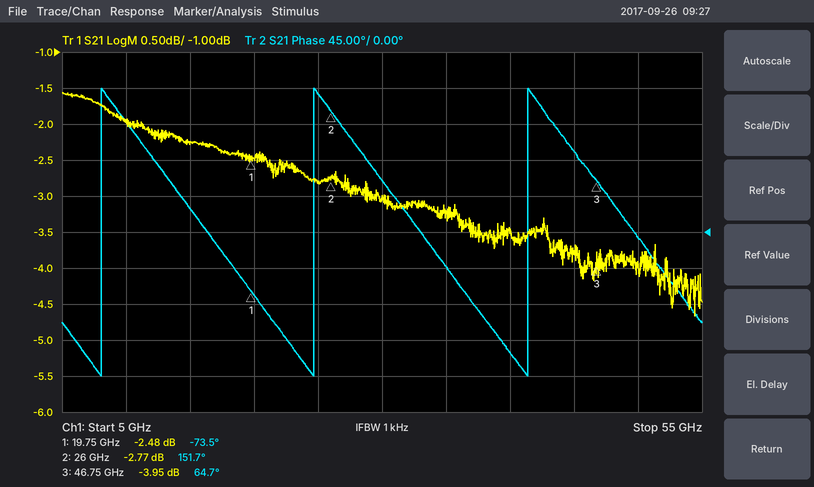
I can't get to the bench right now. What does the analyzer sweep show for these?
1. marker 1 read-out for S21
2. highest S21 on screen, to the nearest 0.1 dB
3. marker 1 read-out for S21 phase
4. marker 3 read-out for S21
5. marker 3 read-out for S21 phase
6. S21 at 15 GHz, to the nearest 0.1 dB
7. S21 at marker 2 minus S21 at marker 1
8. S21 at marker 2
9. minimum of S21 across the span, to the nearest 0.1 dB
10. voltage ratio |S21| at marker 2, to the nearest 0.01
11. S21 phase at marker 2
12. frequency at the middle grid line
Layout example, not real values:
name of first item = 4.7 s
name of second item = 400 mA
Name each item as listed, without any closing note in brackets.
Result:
marker 1 read-out for S21 = -2.48 dB
highest S21 on screen, to the nearest 0.1 dB = -1.6 dB
marker 1 read-out for S21 phase = -73.5°
marker 3 read-out for S21 = -3.95 dB
marker 3 read-out for S21 phase = 64.7°
S21 at 15 GHz, to the nearest 0.1 dB = -2.3 dB
S21 at marker 2 minus S21 at marker 1 = -0.29 dB
S21 at marker 2 = -2.77 dB
minimum of S21 across the span, to the nearest 0.1 dB = -4.7 dB
voltage ratio |S21| at marker 2, to the nearest 0.01 = 0.73
S21 phase at marker 2 = 151.7°
frequency at the middle grid line = 30 GHz
